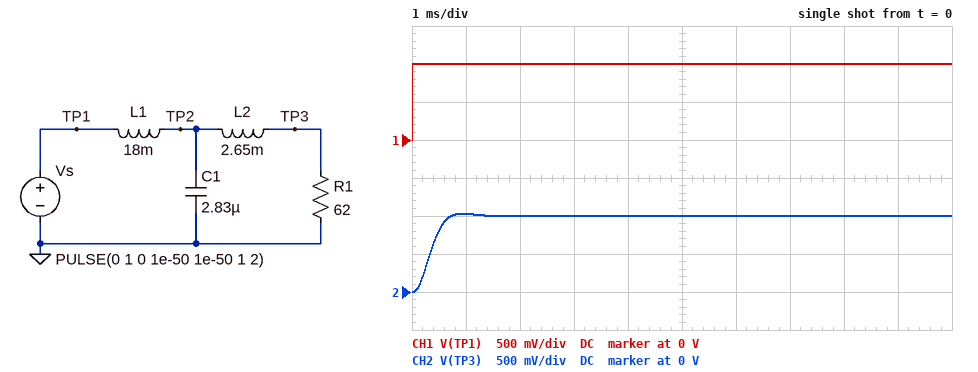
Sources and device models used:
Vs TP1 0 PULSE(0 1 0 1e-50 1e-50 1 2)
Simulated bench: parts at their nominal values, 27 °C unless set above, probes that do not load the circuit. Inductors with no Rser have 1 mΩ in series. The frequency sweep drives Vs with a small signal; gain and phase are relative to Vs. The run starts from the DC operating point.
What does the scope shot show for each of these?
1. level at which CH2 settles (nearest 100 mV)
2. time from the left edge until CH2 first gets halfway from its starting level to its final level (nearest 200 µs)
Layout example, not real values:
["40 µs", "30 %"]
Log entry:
["1.0 V", "400 µs"]
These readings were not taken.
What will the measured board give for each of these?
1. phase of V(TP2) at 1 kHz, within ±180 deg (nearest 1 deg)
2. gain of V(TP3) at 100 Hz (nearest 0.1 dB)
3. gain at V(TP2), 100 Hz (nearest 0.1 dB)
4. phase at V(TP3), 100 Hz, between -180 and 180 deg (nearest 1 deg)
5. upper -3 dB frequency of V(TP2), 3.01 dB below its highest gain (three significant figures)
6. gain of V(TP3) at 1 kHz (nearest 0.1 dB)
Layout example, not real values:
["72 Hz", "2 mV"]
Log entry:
["-108 deg", "0 dB", "0 dB", "-12 deg", "812 Hz", "-5.4 dB"]
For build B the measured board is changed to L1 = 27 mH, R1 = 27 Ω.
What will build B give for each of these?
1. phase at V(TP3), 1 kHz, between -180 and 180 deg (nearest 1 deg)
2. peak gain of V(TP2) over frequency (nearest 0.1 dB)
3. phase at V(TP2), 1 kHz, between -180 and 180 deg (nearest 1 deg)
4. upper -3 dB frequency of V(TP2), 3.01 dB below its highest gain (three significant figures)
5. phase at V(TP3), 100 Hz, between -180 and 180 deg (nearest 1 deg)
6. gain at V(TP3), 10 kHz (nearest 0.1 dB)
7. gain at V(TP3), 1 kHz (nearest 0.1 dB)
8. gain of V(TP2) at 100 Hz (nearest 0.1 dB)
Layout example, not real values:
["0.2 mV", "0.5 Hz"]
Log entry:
["-112 deg", "0 dB", "-80 deg", "157 Hz", "-35 deg", "-65.2 dB", "-14.7 dB", "-1.5 dB"]
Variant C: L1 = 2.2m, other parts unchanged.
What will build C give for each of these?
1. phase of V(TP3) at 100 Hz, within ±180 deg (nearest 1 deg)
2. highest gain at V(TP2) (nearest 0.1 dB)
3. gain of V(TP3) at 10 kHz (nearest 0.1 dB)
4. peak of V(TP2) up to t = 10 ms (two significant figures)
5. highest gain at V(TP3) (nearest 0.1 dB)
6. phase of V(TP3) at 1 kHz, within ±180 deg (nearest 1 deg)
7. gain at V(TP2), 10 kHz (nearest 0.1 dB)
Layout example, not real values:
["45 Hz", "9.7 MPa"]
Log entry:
["-3 deg", "8.8 dB", "-36.3 dB", "1.5 V", "7.5 dB", "-29 deg", "-27.2 dB"]
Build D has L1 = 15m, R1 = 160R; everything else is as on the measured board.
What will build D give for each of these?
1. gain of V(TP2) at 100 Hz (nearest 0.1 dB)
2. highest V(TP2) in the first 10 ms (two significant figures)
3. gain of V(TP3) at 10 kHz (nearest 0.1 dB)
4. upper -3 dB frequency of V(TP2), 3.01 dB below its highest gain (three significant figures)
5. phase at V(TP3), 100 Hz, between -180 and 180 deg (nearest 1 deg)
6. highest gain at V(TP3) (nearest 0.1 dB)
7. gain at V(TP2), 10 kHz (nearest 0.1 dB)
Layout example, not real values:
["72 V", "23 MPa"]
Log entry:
["0.1 dB", "1.5 V", "-47.5 dB", "912 Hz", "-4 deg", "6.9 dB", "-44.3 dB"]
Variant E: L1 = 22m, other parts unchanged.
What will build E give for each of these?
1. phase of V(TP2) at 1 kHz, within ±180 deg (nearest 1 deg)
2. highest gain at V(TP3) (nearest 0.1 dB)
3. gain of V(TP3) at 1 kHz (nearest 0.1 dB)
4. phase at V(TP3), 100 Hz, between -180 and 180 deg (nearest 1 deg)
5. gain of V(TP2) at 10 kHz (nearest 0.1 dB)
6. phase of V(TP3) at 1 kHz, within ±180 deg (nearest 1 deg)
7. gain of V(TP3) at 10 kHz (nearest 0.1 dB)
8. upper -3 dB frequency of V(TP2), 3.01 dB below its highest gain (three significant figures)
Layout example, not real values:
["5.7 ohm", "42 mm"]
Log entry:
["-113 deg", "0 dB", "-7.4 dB", "-14 deg", "-47.5 dB", "-128 deg", "-56.7 dB", "646 Hz"]
